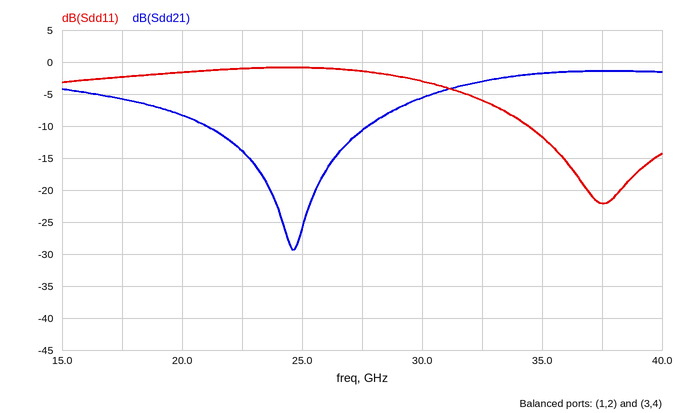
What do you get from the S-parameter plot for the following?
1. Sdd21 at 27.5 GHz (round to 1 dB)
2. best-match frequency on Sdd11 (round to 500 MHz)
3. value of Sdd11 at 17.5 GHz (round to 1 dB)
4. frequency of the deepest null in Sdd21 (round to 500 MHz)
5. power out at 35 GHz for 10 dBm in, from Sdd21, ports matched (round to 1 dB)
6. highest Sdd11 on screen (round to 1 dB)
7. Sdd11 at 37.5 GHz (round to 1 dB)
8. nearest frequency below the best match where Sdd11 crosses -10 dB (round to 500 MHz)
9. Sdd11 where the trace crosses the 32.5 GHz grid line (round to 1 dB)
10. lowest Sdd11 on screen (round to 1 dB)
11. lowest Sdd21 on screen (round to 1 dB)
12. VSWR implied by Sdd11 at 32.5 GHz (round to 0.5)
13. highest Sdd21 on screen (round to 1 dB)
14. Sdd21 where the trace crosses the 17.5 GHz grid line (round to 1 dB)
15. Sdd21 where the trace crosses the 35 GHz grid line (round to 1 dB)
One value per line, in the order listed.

-11 dB
37.5 GHz
-2 dB
24.5 GHz
8 dBm
-1 dB
-22 dB
34.5 GHz
-6 dB
-22 dB
-29 dB
3.0
-1 dB
-6 dB
-2 dB
